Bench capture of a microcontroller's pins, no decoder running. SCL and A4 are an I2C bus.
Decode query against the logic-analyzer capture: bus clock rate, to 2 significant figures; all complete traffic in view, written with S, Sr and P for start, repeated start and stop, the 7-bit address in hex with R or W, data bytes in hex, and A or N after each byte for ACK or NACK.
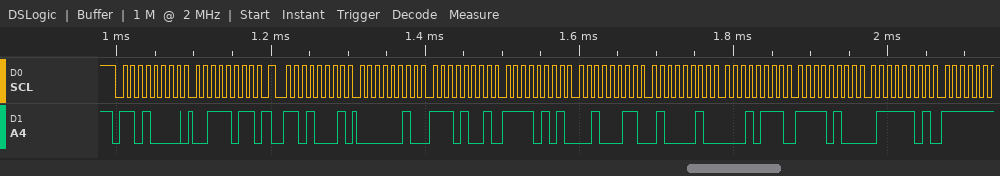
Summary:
100 kHz
S 68W A 3B A Sr 68R A 02 A E9 A F5 A 23 A 42 A 17 A F4 A 7D A
